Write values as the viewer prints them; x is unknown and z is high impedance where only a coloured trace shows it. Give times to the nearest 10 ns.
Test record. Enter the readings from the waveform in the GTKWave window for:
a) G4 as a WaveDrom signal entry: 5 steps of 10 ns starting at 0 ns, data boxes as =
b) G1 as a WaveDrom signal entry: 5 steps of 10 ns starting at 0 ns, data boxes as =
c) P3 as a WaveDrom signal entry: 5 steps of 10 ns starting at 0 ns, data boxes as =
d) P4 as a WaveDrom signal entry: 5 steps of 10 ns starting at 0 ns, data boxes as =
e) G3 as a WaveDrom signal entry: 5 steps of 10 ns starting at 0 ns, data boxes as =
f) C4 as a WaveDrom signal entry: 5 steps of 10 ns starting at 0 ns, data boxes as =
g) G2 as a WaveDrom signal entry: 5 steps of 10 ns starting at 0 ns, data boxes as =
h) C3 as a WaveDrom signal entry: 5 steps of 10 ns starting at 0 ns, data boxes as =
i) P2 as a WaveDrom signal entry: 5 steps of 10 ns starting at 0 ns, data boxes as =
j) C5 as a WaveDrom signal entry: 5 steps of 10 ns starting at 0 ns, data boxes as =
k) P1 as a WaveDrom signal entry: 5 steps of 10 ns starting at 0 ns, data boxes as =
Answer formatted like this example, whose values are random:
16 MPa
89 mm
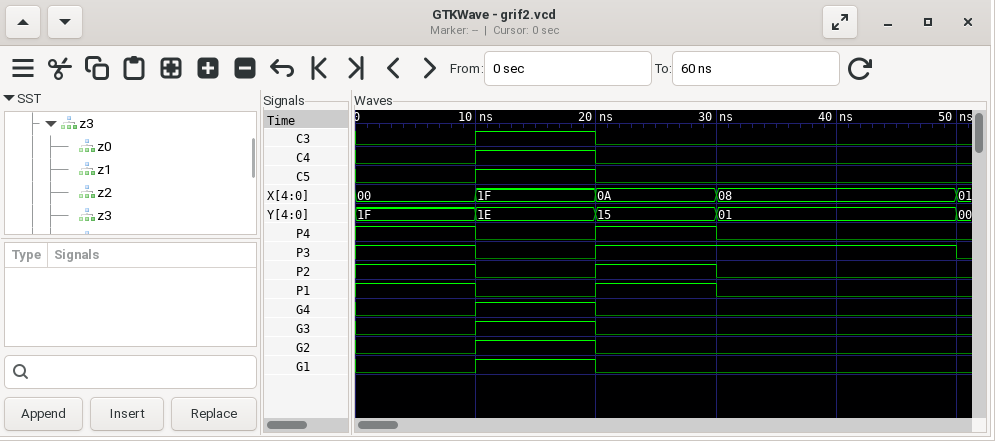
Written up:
{name: 'G4', wave: '010..'}
{name: 'G1', wave: '010..'}
{name: 'P3', wave: '101..'}
{name: 'P4', wave: '1010.'}
{name: 'G3', wave: '010..'}
{name: 'C4', wave: '010..'}
{name: 'G2', wave: '010..'}
{name: 'C3', wave: '010..'}
{name: 'P2', wave: '1010.'}
{name: 'C5', wave: '010..'}
{name: 'P1', wave: '1010.'}
